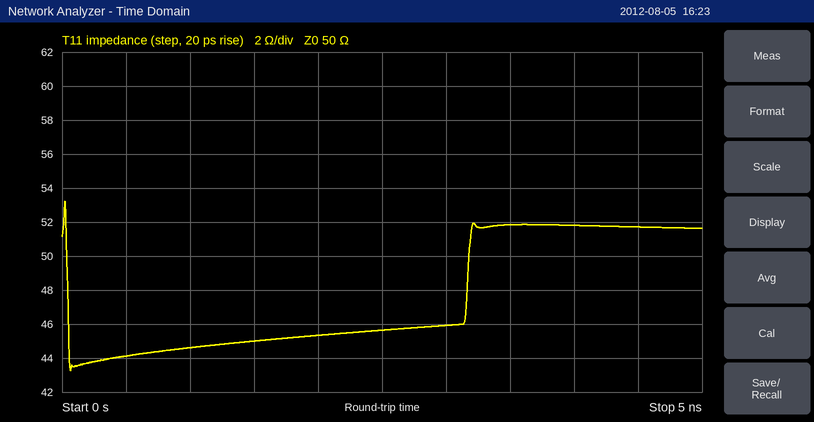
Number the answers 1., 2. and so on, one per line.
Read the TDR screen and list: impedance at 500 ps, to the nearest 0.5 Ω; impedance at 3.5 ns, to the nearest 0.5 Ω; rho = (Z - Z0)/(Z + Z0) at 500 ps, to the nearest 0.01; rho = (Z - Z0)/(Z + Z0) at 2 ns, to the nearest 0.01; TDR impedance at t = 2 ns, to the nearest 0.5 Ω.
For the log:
1. 44.0 Ω
2. 52.0 Ω
3. -0.06
4. -0.05
5. 45.5 Ω
